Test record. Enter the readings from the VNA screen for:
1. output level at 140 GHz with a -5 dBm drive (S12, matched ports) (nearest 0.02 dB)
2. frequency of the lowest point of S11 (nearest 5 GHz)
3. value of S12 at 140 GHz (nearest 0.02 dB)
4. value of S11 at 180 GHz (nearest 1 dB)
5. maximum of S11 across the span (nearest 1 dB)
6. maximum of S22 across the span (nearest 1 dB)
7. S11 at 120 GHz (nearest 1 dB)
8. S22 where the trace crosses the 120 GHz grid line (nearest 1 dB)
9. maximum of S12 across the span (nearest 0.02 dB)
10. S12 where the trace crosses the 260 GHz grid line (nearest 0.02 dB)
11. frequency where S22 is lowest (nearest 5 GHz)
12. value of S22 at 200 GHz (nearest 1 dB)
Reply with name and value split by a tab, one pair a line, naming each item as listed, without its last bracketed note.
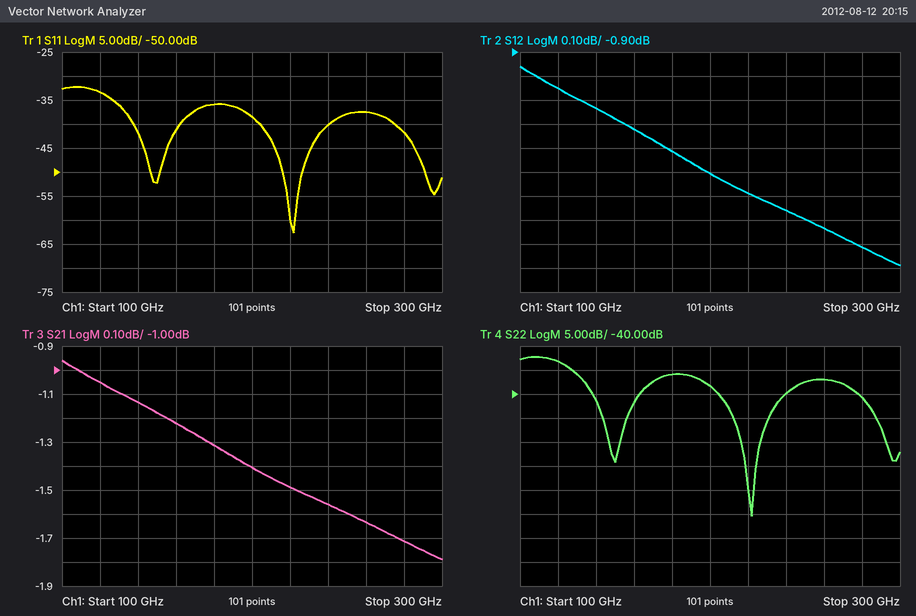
output level at 140 GHz with a -5 dBm drive (S12, matched ports)	-6.14 dBm
frequency of the lowest point of S11	220 GHz
value of S12 at 140 GHz	-1.14 dB
value of S11 at 180 GHz	-36 dB
maximum of S11 across the span	-32 dB
maximum of S22 across the span	-32 dB
S11 at 120 GHz	-33 dB
S22 where the trace crosses the 120 GHz grid line	-33 dB
maximum of S12 across the span	-0.96 dB
S12 where the trace crosses the 260 GHz grid line	-1.64 dB
frequency where S22 is lowest	220 GHz
value of S22 at 200 GHz	-38 dB
